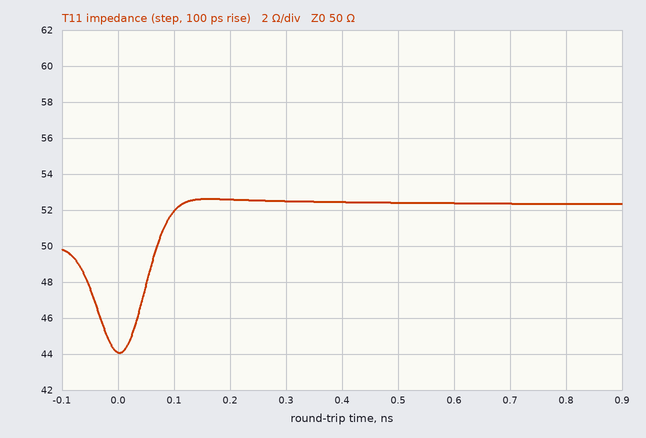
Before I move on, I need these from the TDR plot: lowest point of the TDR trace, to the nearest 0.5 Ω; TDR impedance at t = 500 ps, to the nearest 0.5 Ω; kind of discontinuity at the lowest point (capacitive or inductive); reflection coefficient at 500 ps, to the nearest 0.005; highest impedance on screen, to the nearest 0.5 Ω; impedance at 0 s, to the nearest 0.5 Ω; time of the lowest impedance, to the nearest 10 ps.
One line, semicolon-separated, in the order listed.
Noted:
44.0 Ω; 52.5 Ω; capacitive; +0.025; 52.5 Ω; 44.0 Ω; 0 ps
